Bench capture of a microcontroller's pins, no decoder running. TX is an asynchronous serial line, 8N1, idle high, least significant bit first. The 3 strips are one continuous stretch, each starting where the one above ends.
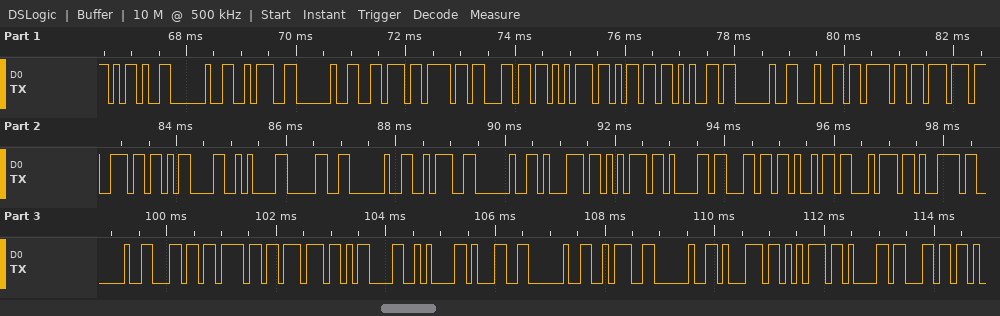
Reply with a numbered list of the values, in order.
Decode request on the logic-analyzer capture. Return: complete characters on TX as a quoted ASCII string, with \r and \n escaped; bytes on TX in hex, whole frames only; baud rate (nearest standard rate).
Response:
1. "- : volume down\r\n0 : quality low\r\n1 : qual"
2. 2D 20 3A 20 76 6F 6C 75 6D 65 20 64 6F 77 6E 0D 0A 30 20 3A 20 71 75 61 6C 69 74 79 20 6C 6F 77 0D 0A 31 20 3A 20 71 75 61 6C
3. 9600 baud
